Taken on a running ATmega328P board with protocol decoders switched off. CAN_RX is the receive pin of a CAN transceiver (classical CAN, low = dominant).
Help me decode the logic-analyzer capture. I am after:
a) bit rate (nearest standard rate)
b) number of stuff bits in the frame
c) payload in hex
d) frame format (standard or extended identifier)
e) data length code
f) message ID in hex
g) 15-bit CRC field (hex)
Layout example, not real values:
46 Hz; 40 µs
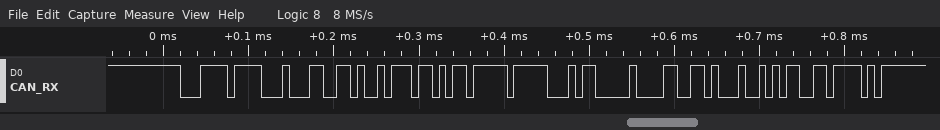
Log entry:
125 kbit/s; 3; CD 2E D6 FF CB 00 66 89; standard; 8; 0x1EF; 0x2CDE
